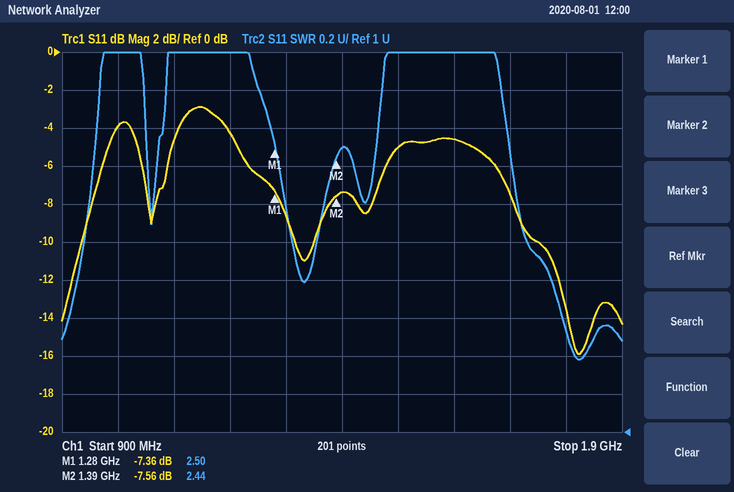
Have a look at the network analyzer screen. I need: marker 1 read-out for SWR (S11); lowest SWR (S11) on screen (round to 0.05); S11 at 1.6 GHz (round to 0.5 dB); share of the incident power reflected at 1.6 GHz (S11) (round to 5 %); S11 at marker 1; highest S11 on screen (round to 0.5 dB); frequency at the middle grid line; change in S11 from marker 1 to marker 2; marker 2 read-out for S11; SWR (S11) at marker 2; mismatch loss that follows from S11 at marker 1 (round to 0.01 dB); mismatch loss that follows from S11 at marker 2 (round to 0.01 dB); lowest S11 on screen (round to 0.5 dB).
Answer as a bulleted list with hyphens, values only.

- 2.50
- 1.40
- -4.5 dB
- 35 %
- -7.36 dB
- -3.0 dB
- 1.4 GHz
- -0.20 dB
- -7.56 dB
- 2.44
- 0.88 dB
- 0.84 dB
- -16.0 dB
